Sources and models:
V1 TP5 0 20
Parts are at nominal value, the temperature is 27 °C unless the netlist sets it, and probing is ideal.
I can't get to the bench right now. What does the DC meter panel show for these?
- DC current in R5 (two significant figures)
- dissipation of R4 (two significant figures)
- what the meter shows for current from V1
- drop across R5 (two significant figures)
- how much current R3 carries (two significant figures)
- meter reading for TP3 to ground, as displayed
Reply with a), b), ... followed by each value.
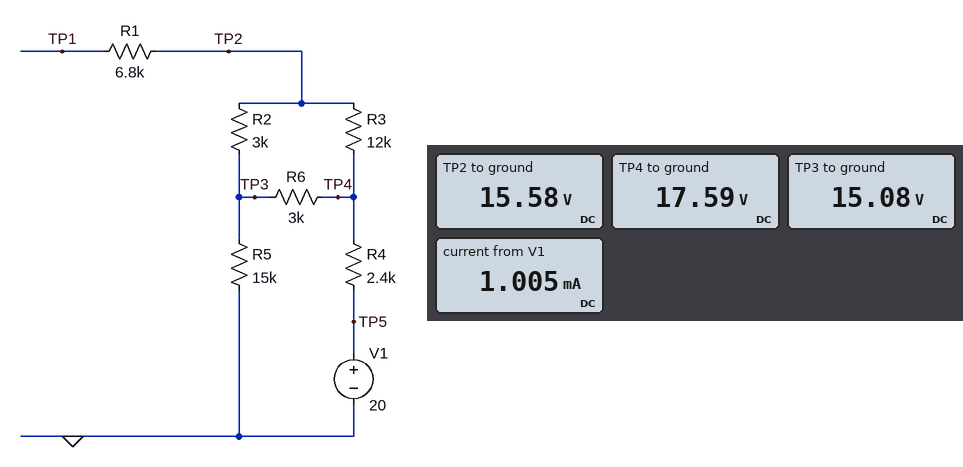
a) 1.0 mA
b) 2.4 mW
c) 1.005 mA
d) 15 V
e) 170 µA
f) 15.08 V
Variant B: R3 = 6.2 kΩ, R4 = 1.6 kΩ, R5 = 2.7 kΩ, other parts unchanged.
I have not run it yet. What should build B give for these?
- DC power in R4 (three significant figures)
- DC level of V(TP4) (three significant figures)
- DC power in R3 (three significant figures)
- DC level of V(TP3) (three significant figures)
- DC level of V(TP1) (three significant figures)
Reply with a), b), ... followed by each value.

a) 14.9 mW
b) 15.1 V
c) 3.48 mW
d) 8.23 V
e) 10.5 V
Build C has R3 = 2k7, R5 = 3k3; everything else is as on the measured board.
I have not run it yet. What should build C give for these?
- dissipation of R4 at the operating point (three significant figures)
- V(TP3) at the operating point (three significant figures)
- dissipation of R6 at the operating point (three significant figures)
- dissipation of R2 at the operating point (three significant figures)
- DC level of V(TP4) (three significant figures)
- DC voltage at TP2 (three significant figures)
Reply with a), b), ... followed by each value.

a) 16.3 mW
b) 8.61 V
c) 8.77 mW
d) 2.43 mW
e) 13.7 V
f) 11.3 V
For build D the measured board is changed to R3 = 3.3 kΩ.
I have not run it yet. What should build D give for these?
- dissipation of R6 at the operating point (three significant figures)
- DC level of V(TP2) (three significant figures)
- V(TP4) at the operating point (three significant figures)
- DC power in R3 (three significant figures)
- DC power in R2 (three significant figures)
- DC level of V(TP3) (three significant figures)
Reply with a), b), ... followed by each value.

a) 1.46 mW
b) 16.4 V
c) 17.5 V
d) 364 µW
e) 331 µW
f) 15.4 V
